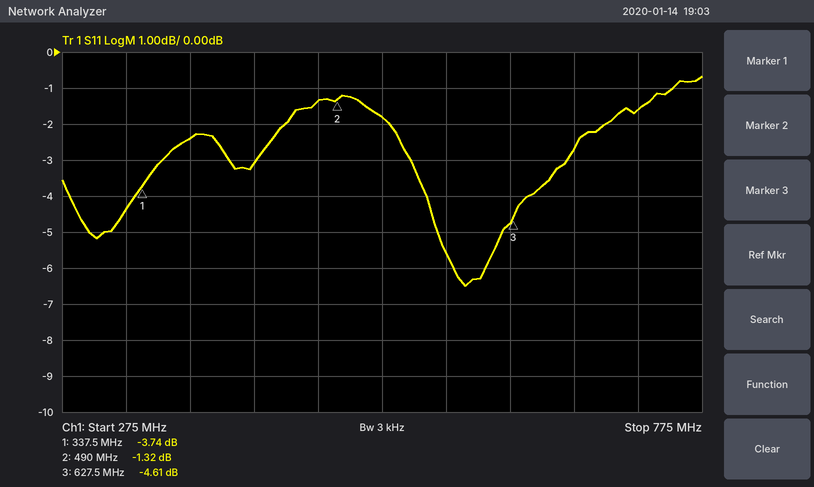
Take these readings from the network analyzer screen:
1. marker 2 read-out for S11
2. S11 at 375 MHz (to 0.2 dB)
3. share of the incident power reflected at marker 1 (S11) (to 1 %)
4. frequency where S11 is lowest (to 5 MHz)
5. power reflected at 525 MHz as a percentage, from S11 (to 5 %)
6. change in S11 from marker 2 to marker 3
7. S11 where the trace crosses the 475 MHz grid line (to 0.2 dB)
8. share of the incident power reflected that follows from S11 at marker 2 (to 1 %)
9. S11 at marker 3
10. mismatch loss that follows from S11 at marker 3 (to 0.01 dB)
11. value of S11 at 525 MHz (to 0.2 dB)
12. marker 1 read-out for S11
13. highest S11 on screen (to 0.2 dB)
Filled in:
-1.32 dB
-2.4 dB
42 %
590 MHz
65 %
-3.29 dB
-1.4 dB
74 %
-4.61 dB
1.84 dB
-1.8 dB
-3.74 dB
-0.6 dB
